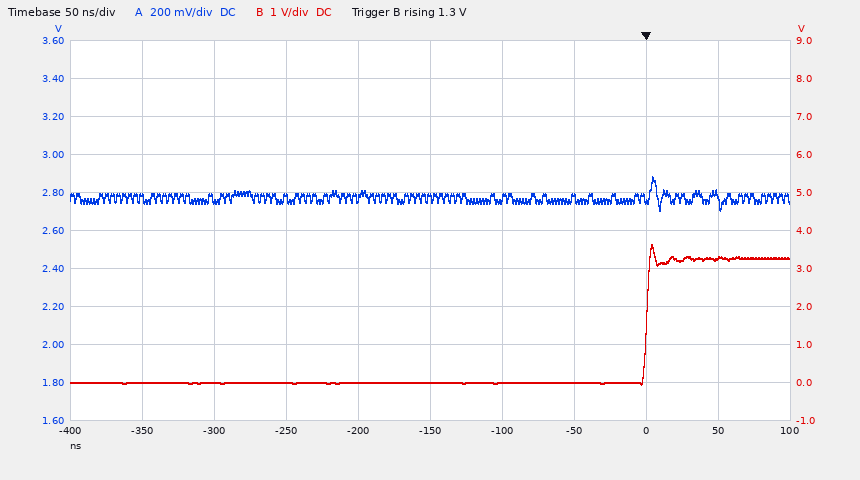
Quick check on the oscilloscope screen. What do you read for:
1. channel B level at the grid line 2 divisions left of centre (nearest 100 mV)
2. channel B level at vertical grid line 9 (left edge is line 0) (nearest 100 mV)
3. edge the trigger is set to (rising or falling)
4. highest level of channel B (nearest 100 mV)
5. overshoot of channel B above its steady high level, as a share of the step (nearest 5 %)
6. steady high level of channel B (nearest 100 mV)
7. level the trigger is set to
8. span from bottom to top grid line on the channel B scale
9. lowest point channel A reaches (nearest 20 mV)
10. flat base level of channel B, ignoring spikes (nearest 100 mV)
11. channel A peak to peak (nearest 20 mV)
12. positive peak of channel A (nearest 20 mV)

0.0 V
3.3 V
rising
3.6 V
10 %
3.3 V
1.3 V
10 V
2.70 V
0.0 V
180 mV
2.88 V
